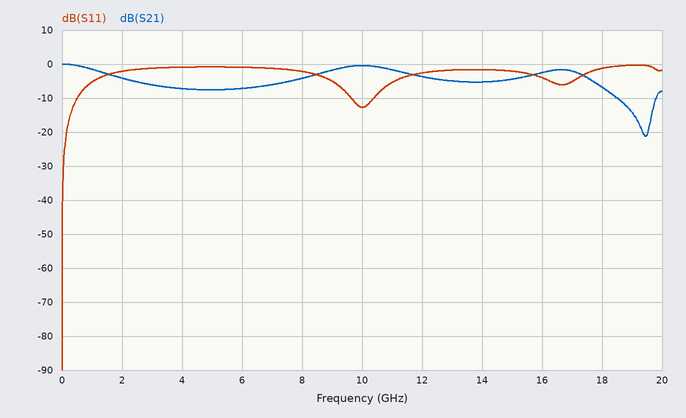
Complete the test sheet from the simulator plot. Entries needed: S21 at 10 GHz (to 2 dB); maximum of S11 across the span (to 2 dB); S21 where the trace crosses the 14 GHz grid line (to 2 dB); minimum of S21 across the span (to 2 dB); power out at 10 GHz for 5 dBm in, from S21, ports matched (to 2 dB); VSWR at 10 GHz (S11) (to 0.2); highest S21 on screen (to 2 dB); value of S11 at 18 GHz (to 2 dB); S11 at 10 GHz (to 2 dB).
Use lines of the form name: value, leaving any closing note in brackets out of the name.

S21 at 10 GHz: 0 dB
maximum of S11 across the span: 0 dB
S21 where the trace crosses the 14 GHz grid line: -6 dB
minimum of S21 across the span: -22 dB
power out at 10 GHz for 5 dBm in, from S21, ports matched: 4 dBm
VSWR at 10 GHz (S11): 1.6
highest S21 on screen: 0 dB
value of S11 at 18 GHz: -2 dB
S11 at 10 GHz: -12 dB
